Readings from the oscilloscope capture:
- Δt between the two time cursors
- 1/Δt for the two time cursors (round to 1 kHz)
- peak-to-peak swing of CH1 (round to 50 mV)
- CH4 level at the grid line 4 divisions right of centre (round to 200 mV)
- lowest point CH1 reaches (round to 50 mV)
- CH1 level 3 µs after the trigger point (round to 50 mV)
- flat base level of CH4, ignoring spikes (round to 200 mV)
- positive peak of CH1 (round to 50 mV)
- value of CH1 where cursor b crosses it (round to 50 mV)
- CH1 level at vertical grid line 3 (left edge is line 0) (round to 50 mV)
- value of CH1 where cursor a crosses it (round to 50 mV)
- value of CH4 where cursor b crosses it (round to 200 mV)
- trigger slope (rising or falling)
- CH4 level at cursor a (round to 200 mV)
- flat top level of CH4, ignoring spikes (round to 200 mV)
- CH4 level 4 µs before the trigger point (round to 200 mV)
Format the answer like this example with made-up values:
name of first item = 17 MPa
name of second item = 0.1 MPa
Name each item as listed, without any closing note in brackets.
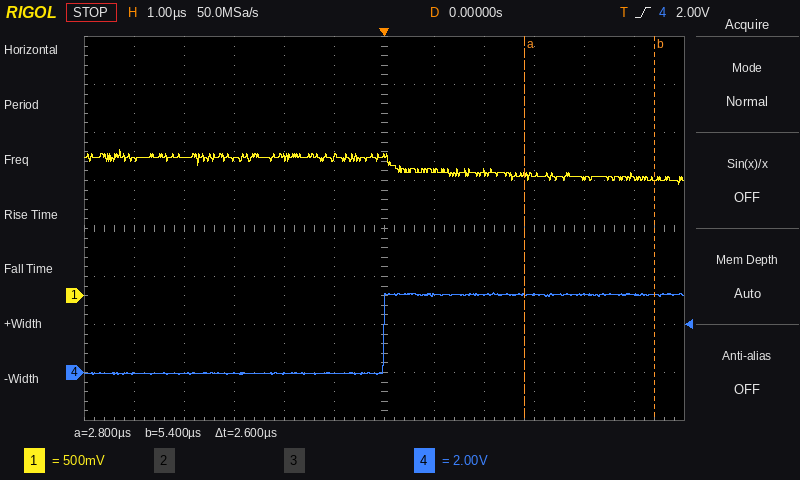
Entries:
Δt between the two time cursors = 2.6 µs
1/Δt for the two time cursors = 385 kHz
peak-to-peak swing of CH1 = 350 mV
CH4 level at the grid line 4 divisions right of centre = 3.2 V
lowest point CH1 reaches = 1.15 V
CH1 level 3 µs after the trigger point = 1.25 V
flat base level of CH4, ignoring spikes = 0.0 V
positive peak of CH1 = 1.50 V
value of CH1 where cursor b crosses it = 1.20 V
CH1 level at vertical grid line 3 (left edge is line 0) = 1.40 V
value of CH1 where cursor a crosses it = 1.25 V
value of CH4 where cursor b crosses it = 3.2 V
trigger slope = rising
CH4 level at cursor a = 3.2 V
flat top level of CH4, ignoring spikes = 3.2 V
CH4 level 4 µs before the trigger point = 0.0 V
